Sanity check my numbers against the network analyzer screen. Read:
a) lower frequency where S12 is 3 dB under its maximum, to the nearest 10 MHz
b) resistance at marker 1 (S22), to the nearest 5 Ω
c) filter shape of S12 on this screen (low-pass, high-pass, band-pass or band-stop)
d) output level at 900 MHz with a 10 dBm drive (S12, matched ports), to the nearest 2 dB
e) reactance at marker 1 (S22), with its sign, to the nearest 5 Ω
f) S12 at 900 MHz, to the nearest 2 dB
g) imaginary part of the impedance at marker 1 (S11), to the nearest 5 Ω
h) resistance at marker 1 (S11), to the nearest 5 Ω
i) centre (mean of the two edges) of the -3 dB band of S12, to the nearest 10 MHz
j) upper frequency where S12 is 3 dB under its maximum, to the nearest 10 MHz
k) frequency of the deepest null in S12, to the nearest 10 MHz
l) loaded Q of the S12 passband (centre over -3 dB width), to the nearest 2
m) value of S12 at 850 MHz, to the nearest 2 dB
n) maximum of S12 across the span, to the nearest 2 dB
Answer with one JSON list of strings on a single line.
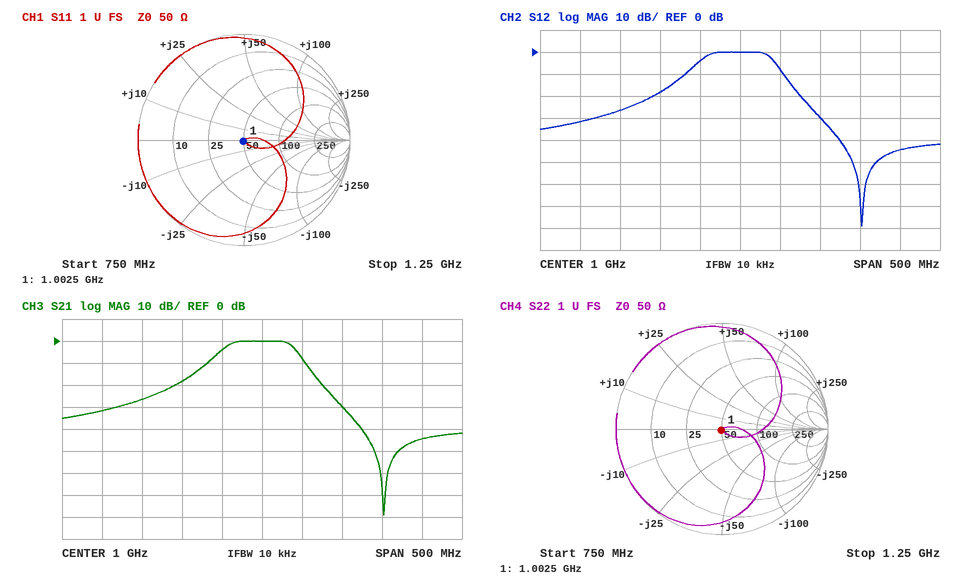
["950 MHz", "50 Ω", "band-pass", "-8 dBm", "0 Ω", "-18 dB", "0 Ω", "50 Ω", "1.00 GHz", "1.04 GHz", "1.15 GHz", "12", "-26 dB", "0 dB"]
